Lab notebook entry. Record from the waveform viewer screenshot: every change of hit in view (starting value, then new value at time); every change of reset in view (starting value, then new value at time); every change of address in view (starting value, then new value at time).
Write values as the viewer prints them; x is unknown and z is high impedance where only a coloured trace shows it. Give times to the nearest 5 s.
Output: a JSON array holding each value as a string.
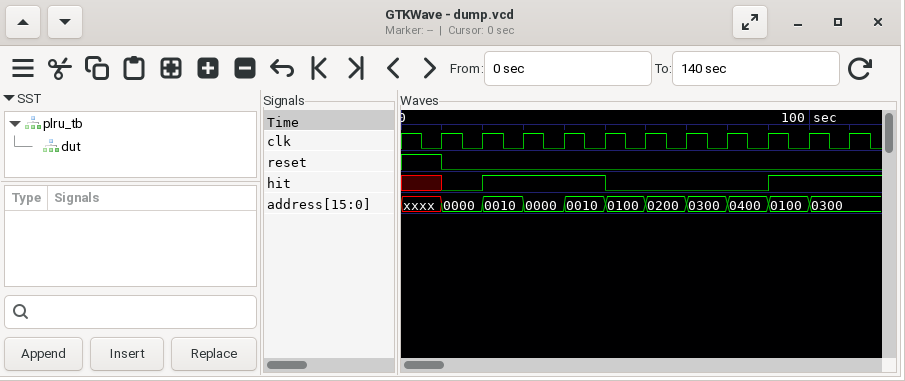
["x, 0 at 10 s, 1 at 20 s, 0 at 50 s, 1 at 90 s", "1, 0 at 10 s", "xxxx, 0000 at 10 s, 0010 at 20 s, 0000 at 30 s, 0010 at 40 s, 0100 at 50 s, 0200 at 60 s, 0300 at 70 s, 0400 at 80 s, 0100 at 90 s, 0300 at 100 s"]
